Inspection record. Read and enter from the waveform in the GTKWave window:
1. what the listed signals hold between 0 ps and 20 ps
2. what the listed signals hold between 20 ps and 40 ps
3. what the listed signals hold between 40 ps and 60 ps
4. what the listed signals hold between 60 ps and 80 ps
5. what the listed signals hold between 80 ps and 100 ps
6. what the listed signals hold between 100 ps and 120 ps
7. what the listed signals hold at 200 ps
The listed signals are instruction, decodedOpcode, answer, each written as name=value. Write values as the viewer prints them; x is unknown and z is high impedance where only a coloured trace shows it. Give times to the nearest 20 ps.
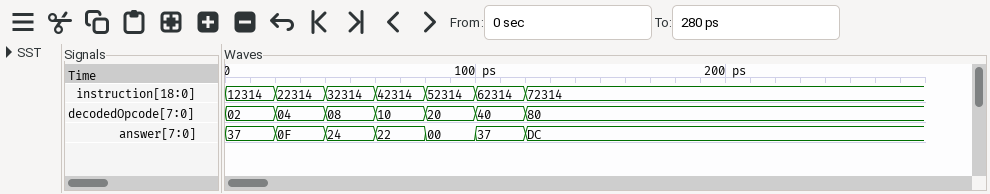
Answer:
instruction=12314, decodedOpcode=02, answer=37
instruction=22314, decodedOpcode=04, answer=0F
instruction=32314, decodedOpcode=08, answer=24
instruction=42314, decodedOpcode=10, answer=22
instruction=52314, decodedOpcode=20, answer=00
instruction=62314, decodedOpcode=40, answer=37
instruction=72314, decodedOpcode=80, answer=DC
